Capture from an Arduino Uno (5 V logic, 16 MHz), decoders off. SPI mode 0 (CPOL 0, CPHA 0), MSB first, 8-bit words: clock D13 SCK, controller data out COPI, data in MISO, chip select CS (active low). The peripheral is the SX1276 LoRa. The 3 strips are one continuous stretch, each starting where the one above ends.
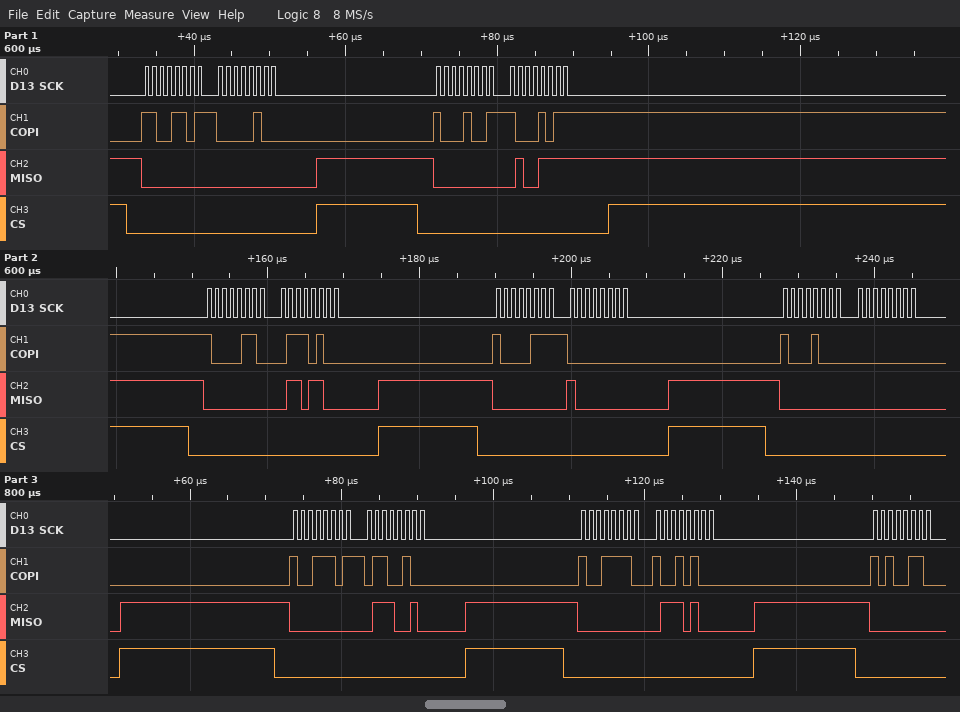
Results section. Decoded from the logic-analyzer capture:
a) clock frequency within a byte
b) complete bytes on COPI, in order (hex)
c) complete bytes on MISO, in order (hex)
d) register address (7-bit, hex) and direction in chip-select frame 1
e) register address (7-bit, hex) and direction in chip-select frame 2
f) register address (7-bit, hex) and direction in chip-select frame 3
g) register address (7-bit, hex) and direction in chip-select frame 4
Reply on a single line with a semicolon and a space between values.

1 MHz; CD 04 89 8B 86 74 87 00 88 00 9D 64 9E 94 A6; 00 00 00 4F 00 6C 00 80 00 00 00 72 00 74 00; 0x4D write; 0x09 write; 0x06 write; 0x07 write
